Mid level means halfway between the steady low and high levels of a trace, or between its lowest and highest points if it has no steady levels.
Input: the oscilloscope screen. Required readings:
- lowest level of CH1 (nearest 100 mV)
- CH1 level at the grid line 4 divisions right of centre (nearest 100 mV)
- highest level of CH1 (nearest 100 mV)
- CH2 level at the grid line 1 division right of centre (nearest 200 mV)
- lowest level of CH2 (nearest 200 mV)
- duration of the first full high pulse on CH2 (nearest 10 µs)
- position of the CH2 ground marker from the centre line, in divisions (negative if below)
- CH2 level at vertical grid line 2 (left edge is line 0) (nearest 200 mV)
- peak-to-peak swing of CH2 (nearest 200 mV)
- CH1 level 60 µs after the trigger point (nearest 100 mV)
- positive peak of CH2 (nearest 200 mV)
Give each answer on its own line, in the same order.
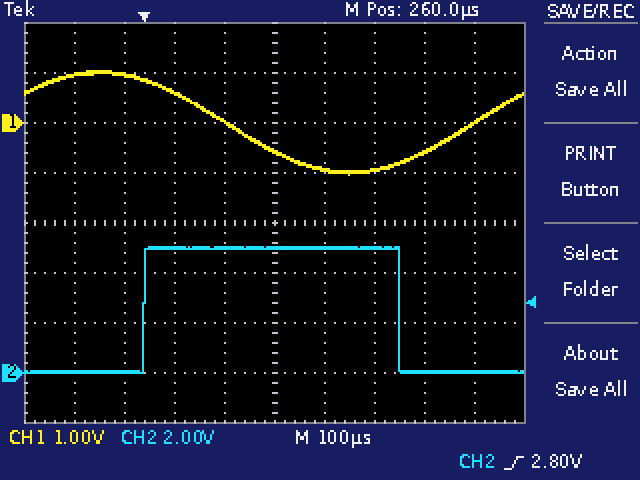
-1.0 V
0.0 V
1.0 V
5.0 V
0.0 V
510 µs
-3.0 div
0.0 V
5.0 V
600 mV
5.0 V
